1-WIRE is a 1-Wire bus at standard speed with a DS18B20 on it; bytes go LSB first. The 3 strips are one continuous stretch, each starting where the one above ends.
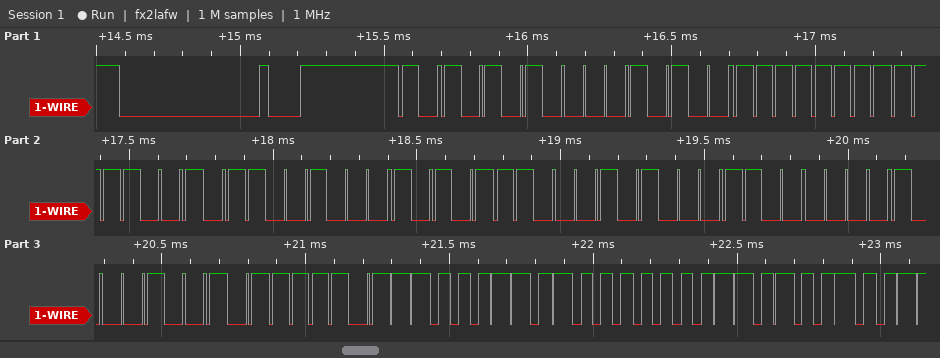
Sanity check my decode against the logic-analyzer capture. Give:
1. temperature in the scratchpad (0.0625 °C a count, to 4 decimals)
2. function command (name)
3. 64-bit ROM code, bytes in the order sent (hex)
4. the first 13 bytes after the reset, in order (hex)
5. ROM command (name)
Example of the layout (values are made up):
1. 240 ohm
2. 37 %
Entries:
1. 22.1875 °C
2. Read Scratchpad
3. 28 FF 4F 13 75 14 03 91
4. 55 28 FF 4F 13 75 14 03 91 BE 63 01 4B
5. Match ROM
